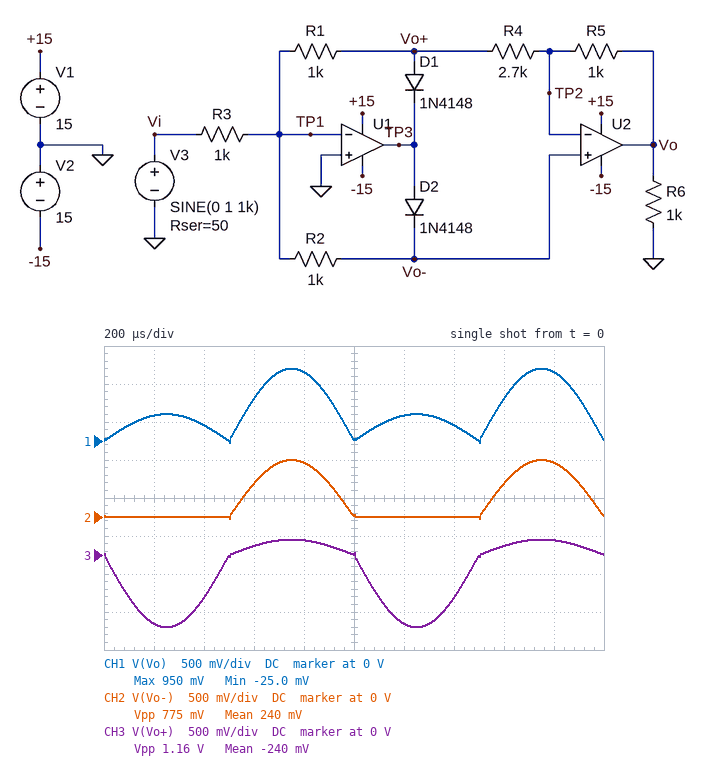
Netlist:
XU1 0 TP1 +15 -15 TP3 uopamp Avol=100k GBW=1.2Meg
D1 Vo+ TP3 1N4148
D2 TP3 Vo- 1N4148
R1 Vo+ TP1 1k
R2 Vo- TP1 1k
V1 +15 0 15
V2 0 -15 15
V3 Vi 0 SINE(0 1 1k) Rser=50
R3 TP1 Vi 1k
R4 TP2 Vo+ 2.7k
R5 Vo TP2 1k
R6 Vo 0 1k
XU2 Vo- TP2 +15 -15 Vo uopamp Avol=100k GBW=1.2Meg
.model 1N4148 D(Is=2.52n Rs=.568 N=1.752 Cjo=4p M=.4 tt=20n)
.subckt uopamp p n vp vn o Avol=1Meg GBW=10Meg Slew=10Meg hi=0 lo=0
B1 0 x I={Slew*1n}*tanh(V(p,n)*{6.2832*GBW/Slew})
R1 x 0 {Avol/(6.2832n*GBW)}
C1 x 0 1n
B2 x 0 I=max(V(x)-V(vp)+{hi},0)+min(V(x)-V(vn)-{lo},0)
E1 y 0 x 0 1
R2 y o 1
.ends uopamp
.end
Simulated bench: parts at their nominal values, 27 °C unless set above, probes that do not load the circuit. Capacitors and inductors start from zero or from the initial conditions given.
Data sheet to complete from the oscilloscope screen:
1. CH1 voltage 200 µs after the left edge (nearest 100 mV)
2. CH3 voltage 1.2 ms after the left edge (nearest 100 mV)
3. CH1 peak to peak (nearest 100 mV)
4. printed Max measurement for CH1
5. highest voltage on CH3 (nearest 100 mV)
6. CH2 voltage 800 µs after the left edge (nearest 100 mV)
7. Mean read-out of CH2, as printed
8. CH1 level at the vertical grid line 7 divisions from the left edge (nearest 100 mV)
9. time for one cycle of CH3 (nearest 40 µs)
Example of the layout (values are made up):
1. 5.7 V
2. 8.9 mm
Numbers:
1. 300 mV
2. -900 mV
3. 1.0 V
4. 950 mV
5. 200 mV
6. 700 mV
7. 240 mV
8. 200 mV
9. 1.00 ms
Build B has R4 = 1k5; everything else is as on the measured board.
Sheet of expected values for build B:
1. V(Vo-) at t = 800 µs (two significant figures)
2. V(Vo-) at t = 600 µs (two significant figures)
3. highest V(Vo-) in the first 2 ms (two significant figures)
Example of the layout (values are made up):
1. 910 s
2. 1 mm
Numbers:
1. 650 mV
2. 400 mV
3. 680 mV
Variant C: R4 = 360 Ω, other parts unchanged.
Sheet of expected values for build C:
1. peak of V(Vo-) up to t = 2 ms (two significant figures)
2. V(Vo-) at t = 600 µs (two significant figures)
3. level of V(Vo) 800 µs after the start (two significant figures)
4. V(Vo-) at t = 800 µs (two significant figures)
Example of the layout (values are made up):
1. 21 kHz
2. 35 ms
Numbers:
1. 550 mV
2. 320 mV
3. 910 mV
4. 520 mV
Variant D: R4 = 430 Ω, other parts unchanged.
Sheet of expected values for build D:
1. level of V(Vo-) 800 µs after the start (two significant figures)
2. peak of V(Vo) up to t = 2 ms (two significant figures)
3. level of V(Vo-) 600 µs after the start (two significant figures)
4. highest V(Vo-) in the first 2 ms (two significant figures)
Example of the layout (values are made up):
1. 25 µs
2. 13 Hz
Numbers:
1. 530 mV
2. 2.2 V
3. 330 mV
4. 560 mV
